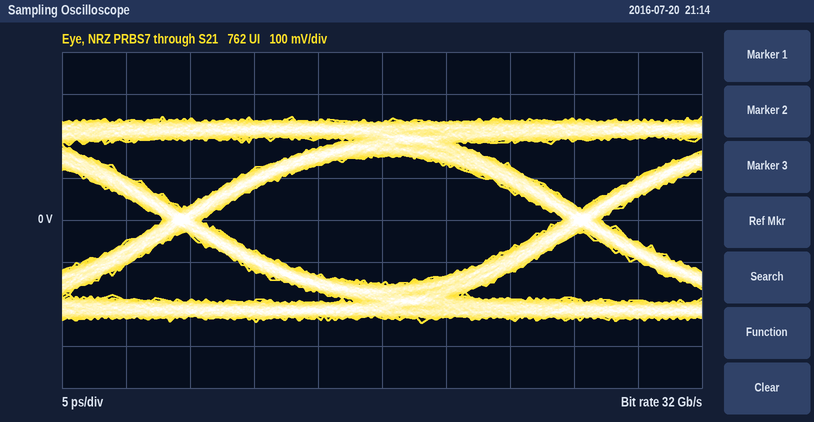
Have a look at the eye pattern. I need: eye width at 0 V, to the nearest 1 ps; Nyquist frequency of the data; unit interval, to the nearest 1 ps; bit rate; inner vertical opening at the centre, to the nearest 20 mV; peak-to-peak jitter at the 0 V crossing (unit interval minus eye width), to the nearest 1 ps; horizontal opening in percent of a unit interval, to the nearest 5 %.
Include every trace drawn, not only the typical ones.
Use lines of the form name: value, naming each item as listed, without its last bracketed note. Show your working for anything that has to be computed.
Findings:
eye width at 0 V, to the nearest 1 ps: 28 ps
Nyquist frequency of the data: 16 GHz
unit interval, to the nearest 1 ps: 31 ps
bit rate: 32 Gb/s
inner vertical opening at the centre, to the nearest 20 mV: 300 mV
peak-to-peak jitter at the 0 V crossing (unit interval minus eye width), to the nearest 1 ps: 3 ps
horizontal opening in percent of a unit interval, to the nearest 5 %: 28 ps / 31 ps ≈ 90 %
